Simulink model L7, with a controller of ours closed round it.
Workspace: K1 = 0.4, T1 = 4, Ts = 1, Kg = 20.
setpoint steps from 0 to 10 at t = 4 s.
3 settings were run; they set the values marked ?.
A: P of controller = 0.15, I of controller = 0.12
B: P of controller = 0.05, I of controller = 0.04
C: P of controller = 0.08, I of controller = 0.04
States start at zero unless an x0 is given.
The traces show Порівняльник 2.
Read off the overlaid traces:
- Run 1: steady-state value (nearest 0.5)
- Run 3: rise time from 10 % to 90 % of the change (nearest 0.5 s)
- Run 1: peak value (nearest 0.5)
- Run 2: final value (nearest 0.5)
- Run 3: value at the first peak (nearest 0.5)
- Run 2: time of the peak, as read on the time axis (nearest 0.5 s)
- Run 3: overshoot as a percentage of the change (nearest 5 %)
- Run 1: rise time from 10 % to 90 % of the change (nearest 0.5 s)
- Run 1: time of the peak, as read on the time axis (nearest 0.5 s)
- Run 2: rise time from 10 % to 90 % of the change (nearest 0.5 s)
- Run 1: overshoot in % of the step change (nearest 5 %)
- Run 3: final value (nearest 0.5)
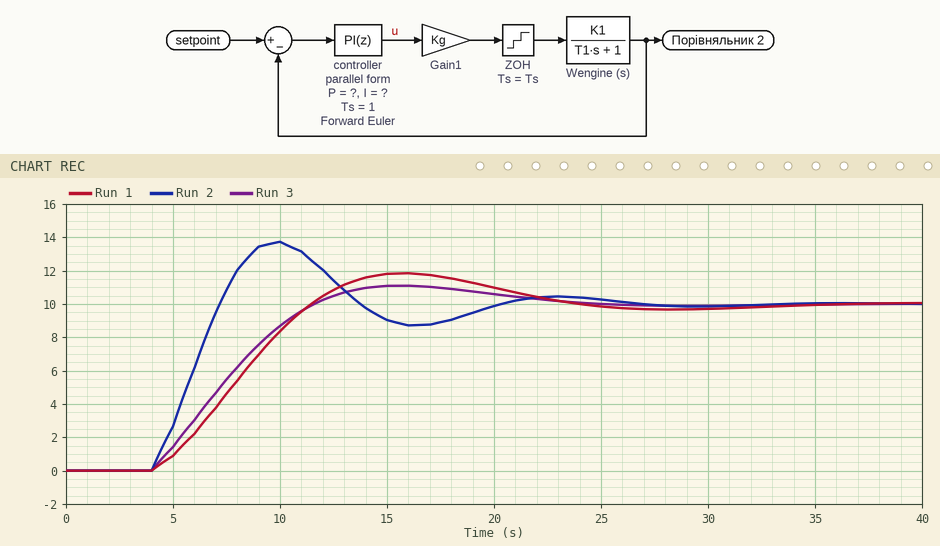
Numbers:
10.0
5.5 s
12.0
10.0
11.0
10.0 s
10 %
5.5 s
16.0 s
2.5 s
20 %
10.0
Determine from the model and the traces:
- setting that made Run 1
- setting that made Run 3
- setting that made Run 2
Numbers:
B
C
A
